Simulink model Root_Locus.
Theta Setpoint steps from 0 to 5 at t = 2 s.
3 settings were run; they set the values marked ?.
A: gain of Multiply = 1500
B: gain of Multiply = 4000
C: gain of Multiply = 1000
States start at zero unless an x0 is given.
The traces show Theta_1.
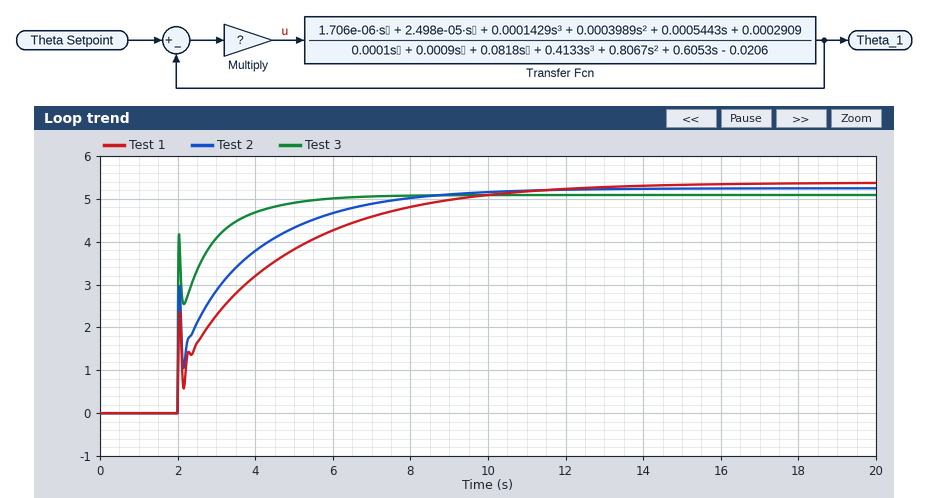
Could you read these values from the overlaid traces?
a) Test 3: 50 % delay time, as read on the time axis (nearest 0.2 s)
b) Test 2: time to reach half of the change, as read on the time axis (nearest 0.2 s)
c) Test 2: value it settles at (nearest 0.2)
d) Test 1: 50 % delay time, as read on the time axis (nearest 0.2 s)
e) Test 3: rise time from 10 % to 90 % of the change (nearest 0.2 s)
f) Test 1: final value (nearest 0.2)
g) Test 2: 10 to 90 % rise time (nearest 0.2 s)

2.0 s
2.0 s
5.2
3.4 s
1.8 s
5.4
4.2 s
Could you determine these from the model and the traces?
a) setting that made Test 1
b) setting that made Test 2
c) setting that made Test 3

C
A
B
